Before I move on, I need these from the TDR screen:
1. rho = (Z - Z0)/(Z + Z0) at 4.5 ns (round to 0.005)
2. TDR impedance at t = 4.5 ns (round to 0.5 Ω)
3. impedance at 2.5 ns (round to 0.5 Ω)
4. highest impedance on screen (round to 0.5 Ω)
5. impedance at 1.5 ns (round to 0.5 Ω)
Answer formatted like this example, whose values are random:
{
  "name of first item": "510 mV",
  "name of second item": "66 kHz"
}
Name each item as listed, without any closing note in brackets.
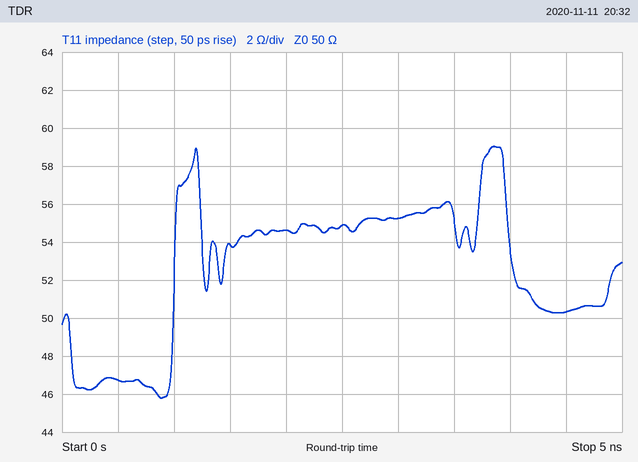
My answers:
{
  "rho = (Z - Z0)/(Z + Z0) at 4.5 ns": "+0.005",
  "TDR impedance at t = 4.5 ns": "50.5 Ω",
  "impedance at 2.5 ns": "55.0 Ω",
  "highest impedance on screen": "59.0 Ω",
  "impedance at 1.5 ns": "54.0 Ω"
}
